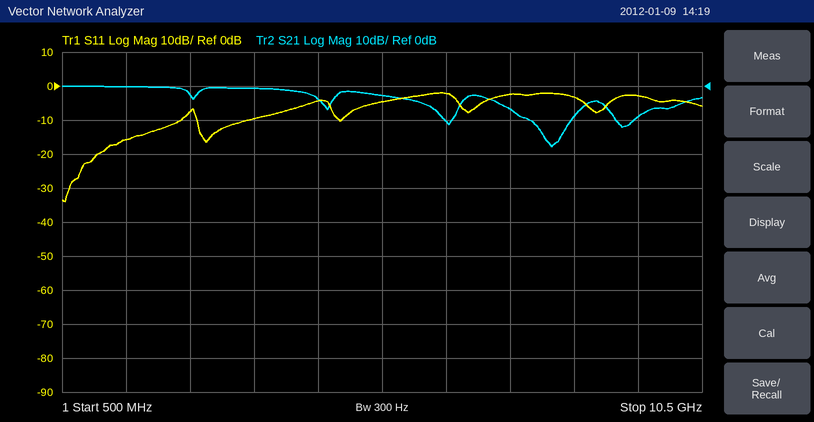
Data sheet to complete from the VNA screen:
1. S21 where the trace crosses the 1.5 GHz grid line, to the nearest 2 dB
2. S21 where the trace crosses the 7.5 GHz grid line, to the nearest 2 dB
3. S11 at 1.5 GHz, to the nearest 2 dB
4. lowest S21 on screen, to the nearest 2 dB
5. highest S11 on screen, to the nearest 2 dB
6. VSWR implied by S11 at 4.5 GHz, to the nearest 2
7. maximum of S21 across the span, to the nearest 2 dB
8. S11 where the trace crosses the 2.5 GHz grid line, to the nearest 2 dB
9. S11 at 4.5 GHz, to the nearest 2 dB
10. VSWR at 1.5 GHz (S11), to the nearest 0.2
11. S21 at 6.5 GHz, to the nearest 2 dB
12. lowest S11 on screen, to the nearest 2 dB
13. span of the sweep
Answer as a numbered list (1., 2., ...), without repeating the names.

1. 0 dB
2. -6 dB
3. -16 dB
4. -18 dB
5. -2 dB
6. 4
7. 0 dB
8. -8 dB
9. -4 dB
10. 1.4
11. -10 dB
12. -34 dB
13. 10 GHz
